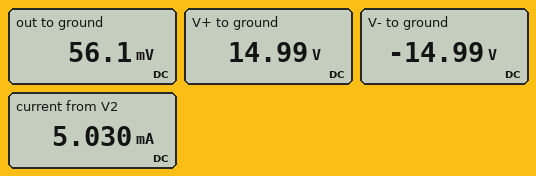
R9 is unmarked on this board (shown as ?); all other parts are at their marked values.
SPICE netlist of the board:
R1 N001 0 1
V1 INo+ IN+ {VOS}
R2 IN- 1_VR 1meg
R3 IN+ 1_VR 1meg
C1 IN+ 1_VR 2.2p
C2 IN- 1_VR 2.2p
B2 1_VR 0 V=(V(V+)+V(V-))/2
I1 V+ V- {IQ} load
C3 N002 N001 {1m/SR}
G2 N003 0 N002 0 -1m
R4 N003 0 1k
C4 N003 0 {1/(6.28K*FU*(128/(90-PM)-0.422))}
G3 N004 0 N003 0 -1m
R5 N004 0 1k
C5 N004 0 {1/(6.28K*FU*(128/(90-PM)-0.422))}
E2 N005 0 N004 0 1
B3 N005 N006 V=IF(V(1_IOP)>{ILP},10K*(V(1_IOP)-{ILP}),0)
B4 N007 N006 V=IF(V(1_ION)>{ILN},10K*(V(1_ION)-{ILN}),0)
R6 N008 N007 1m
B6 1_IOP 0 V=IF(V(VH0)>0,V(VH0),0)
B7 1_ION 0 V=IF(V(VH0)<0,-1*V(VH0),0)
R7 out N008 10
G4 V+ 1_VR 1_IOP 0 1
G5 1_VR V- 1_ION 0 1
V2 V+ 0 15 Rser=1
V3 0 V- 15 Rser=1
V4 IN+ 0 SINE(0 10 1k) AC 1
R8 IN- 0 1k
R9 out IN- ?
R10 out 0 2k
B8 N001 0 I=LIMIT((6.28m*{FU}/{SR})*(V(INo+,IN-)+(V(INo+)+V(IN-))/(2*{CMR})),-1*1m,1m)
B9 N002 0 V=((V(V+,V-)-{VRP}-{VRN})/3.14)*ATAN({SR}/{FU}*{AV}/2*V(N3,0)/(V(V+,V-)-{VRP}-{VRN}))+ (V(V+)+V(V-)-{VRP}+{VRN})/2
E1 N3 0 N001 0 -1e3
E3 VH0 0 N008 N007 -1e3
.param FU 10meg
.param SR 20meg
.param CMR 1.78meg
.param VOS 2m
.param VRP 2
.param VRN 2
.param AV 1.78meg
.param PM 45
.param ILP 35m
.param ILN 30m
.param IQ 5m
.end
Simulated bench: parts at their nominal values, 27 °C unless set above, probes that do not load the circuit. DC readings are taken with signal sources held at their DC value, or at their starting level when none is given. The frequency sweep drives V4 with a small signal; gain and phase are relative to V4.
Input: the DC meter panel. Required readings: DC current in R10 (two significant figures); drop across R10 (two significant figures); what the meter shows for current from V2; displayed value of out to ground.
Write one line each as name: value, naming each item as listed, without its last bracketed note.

DC current in R10: 28 µA
drop across R10: 56 mV
what the meter shows for current from V2: 5.030 mA
displayed value of out to ground: 56.1 mV
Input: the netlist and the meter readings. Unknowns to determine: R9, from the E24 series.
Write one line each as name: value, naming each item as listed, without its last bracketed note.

R9, from the E24 series: 27 kΩ
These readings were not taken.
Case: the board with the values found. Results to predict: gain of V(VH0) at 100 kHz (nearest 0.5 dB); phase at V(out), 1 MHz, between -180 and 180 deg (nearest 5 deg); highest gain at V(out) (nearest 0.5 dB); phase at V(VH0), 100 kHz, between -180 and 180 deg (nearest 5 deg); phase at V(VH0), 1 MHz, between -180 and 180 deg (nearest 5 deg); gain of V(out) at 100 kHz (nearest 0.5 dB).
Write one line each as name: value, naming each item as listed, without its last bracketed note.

gain of V(VH0) at 100 kHz: -37.0 dB
phase at V(out), 1 MHz, between -180 and 180 deg: -75 deg
highest gain at V(out): 29.0 dB
phase at V(VH0), 100 kHz, between -180 and 180 deg: -15 deg
phase at V(VH0), 1 MHz, between -180 and 180 deg: -75 deg
gain of V(out) at 100 kHz: 28.5 dB
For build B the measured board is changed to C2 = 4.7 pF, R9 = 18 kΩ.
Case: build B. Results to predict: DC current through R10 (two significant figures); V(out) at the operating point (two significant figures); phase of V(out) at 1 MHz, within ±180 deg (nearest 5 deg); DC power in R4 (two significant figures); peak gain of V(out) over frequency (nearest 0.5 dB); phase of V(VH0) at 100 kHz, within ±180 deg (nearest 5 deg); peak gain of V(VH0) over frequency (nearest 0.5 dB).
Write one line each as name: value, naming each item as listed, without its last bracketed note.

DC current through R10: 19 µA
V(out) at the operating point: 38 mV
phase of V(out) at 1 MHz, within ±180 deg: -65 deg
DC power in R4: 1.5 µW
peak gain of V(out) over frequency: 25.5 dB
phase of V(VH0) at 100 kHz, within ±180 deg: -10 deg
peak gain of V(VH0) over frequency: -39.5 dB
